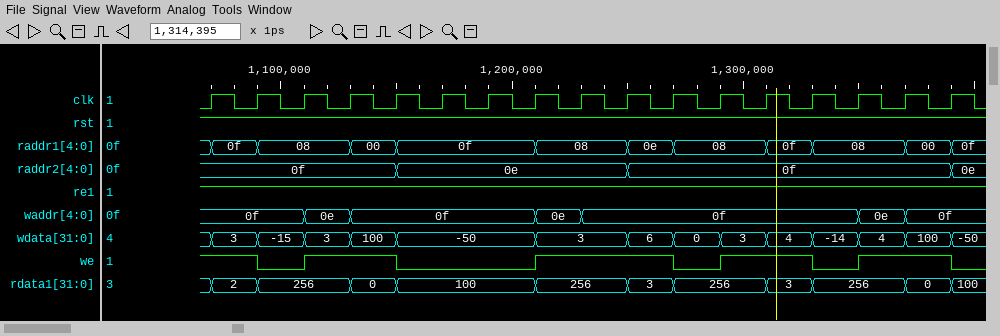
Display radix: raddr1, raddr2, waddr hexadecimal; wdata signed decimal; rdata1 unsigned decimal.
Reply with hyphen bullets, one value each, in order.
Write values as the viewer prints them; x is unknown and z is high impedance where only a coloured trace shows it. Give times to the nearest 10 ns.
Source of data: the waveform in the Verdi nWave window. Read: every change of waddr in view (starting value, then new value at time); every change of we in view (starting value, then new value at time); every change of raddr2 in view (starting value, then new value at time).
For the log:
- 0f, 0e at 1110 ns, 0f at 1130 ns, 0e at 1210 ns, 0f at 1230 ns, 0e at 1350 ns, 0f at 1370 ns
- 1, 0 at 1090 ns, 1 at 1110 ns, 0 at 1150 ns, 1 at 1210 ns, 0 at 1270 ns, 1 at 1290 ns, 0 at 1330 ns, 1 at 1350 ns, 0 at 1390 ns
- 0f, 0e at 1150 ns, 0f at 1250 ns, 0e at 1390 ns
